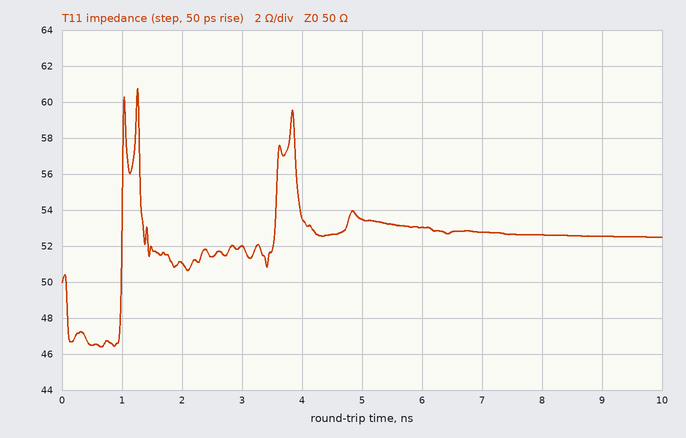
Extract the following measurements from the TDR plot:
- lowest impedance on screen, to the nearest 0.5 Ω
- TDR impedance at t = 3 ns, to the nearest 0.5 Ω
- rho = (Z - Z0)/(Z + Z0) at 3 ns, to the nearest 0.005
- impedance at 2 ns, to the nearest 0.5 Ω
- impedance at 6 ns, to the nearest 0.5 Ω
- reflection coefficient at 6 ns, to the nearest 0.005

46.5 Ω
52.0 Ω
+0.020
51.0 Ω
53.0 Ω
+0.030
